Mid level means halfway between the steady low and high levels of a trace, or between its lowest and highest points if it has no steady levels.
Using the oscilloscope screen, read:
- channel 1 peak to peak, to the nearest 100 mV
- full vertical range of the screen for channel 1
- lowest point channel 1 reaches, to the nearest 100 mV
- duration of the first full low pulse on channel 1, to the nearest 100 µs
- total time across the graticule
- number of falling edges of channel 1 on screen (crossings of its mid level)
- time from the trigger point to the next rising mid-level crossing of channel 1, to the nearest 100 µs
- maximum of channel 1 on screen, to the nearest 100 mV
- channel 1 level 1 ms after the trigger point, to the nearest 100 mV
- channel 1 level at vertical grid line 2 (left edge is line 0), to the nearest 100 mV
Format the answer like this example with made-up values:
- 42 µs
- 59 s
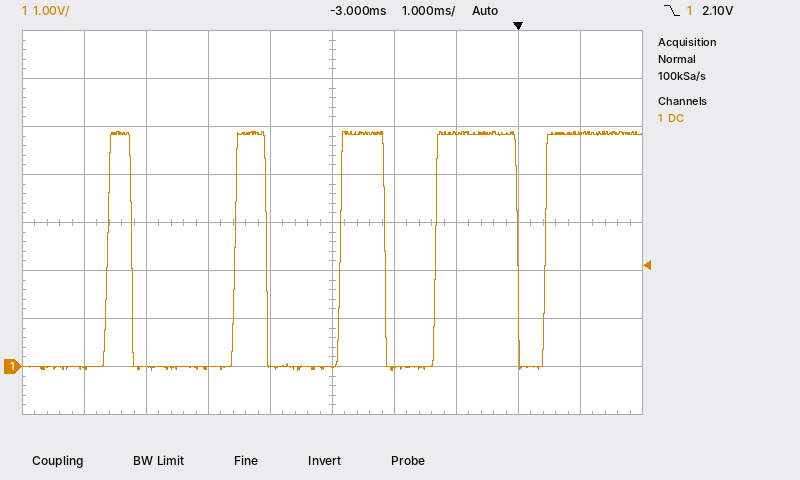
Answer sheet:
- 5.0 V
- 8 V
- -100 mV
- 1.7 ms
- 10 ms
- 4
- 400 µs
- 4.9 V
- 4.9 V
- 0.0 V
